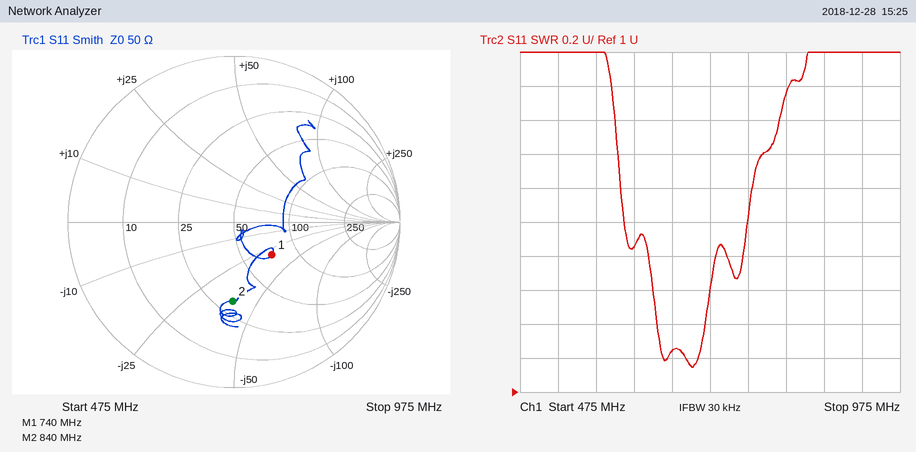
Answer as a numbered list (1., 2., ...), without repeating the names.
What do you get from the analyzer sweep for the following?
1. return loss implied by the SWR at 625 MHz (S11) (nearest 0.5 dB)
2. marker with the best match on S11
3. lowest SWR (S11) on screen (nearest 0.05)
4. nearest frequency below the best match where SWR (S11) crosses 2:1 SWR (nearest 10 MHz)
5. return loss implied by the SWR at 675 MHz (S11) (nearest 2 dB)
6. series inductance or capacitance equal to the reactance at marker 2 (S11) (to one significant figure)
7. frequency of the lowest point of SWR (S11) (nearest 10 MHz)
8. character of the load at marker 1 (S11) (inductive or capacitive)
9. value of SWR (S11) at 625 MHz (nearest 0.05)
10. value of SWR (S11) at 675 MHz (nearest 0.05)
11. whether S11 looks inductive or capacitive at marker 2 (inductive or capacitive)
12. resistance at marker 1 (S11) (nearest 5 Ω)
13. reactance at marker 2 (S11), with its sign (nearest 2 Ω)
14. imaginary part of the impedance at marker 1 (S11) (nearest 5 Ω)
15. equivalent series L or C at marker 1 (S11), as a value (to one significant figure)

1. 10.5 dB
2. marker 1
3. 1.15
4. 610 MHz
5. 20 dB
6. 5 pF
7. 700 MHz
8. capacitive
9. 1.85
10. 1.25
11. capacitive
12. 70 Ω
13. -38 Ω
14. -30 Ω
15. 7 pF
